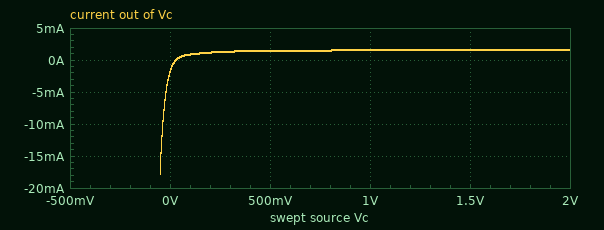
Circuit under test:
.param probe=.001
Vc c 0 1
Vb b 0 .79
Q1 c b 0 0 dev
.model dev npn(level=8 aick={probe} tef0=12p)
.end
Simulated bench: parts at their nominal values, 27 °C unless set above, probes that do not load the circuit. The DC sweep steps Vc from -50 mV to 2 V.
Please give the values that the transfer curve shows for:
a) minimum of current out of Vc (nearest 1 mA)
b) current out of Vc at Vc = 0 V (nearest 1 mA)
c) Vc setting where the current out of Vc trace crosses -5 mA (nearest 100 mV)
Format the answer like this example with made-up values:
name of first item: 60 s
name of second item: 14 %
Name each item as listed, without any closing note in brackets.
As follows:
minimum of current out of Vc: -18 mA
current out of Vc at Vc = 0 V: -2 mA
Vc setting where the current out of Vc trace crosses -5 mA: 0 V
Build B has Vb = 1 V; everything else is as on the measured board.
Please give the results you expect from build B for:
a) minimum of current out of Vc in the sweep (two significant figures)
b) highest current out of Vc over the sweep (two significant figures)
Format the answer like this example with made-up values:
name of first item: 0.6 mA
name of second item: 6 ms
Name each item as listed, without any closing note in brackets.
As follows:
minimum of current out of Vc in the sweep: -43 A
highest current out of Vc over the sweep: 41 mA
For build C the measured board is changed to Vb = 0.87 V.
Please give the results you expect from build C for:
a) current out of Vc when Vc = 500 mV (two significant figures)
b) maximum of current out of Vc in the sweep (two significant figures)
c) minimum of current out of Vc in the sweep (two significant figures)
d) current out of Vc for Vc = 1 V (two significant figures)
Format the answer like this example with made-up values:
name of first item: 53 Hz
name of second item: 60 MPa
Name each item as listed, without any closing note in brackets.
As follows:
current out of Vc when Vc = 500 mV: 6.2 mA
maximum of current out of Vc in the sweep: 7.2 mA
minimum of current out of Vc in the sweep: -300 mA
current out of Vc for Vc = 1 V: 6.9 mA
